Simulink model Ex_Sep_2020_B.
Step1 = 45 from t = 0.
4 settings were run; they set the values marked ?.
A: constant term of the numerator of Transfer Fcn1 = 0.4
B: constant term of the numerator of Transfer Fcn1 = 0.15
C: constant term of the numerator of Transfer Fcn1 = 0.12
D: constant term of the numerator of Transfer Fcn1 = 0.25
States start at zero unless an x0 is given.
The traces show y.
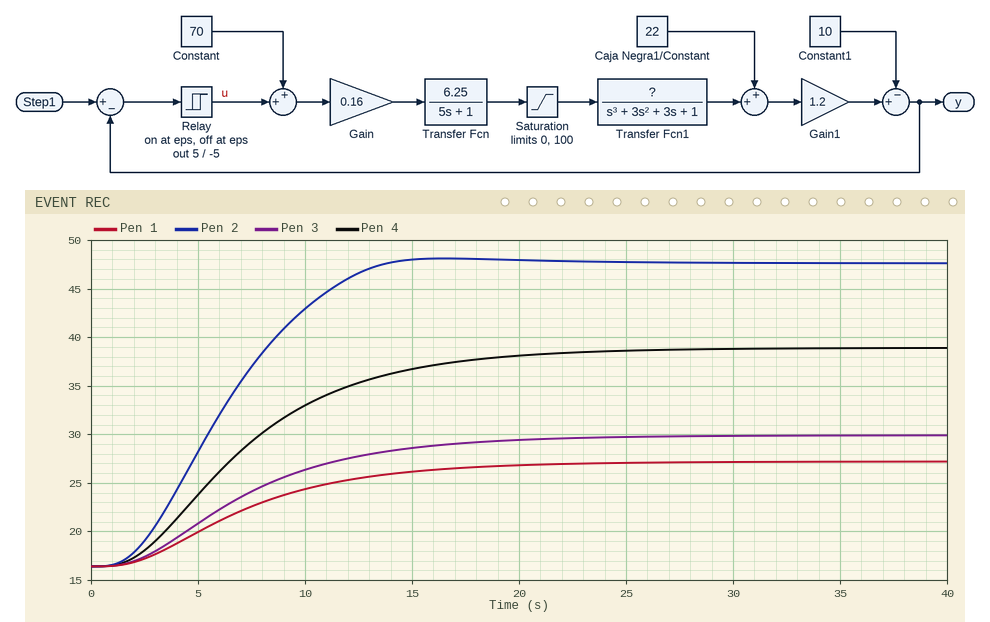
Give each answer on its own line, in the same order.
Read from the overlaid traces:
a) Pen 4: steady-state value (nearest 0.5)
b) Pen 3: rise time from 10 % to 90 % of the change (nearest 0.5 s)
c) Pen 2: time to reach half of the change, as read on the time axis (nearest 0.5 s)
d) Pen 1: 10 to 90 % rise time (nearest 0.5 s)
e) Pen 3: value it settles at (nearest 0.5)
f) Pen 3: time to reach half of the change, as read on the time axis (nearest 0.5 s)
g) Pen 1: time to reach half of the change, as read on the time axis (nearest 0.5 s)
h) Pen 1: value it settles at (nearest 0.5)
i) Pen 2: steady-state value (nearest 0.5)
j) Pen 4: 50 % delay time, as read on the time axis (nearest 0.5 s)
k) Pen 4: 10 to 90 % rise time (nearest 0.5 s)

39.0
12.0 s
6.0 s
12.0 s
30.0
6.5 s
6.5 s
27.0
47.5
6.5 s
12.0 s
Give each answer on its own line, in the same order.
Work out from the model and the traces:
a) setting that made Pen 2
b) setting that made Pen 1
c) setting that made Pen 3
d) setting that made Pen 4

A
C
B
D
